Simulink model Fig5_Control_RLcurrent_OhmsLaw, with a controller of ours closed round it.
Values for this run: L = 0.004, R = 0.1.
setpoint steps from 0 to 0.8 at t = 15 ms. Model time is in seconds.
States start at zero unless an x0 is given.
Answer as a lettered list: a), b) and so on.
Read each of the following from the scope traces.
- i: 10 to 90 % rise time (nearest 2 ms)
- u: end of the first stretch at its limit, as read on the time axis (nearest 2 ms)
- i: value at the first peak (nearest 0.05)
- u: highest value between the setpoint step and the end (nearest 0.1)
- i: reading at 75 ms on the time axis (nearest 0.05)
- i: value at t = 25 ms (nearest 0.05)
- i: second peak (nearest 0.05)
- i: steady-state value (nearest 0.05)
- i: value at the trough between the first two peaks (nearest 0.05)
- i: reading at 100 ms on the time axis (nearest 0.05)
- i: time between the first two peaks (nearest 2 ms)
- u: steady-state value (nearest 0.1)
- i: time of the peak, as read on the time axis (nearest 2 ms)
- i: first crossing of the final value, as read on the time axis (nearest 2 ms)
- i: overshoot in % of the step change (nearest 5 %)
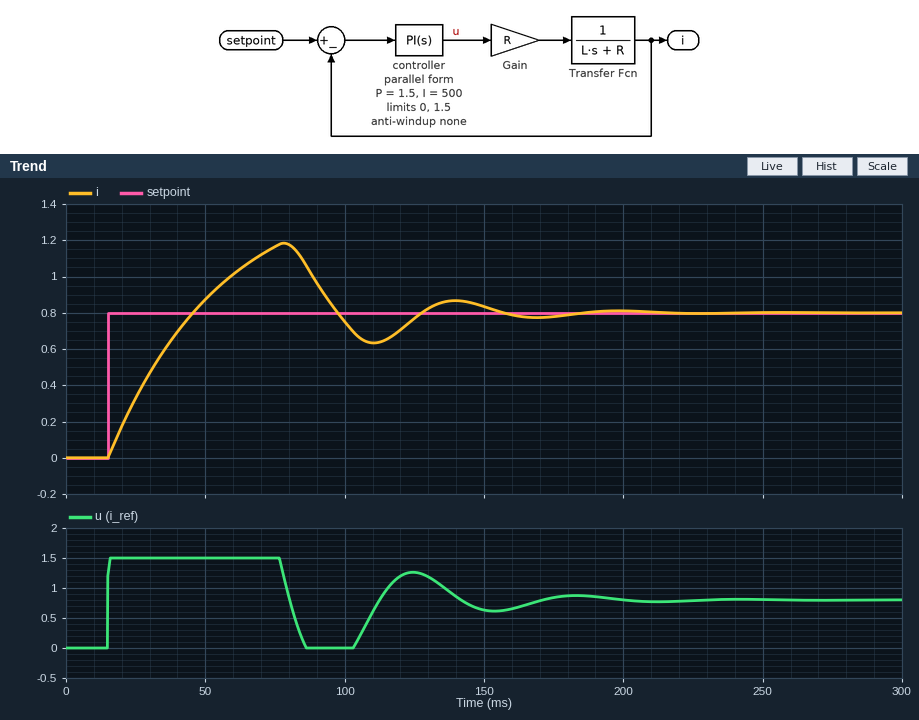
a) 24 ms
b) 76 ms
c) 1.20
d) 1.5
e) 1.15
f) 0.35
g) 0.85
h) 0.80
i) 0.65
j) 0.75
k) 62 ms
l) 0.8
m) 78 ms
n) 46 ms
o) 50 %
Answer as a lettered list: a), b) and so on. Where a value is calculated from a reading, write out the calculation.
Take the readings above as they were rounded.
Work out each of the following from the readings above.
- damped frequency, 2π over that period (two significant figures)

a) 2π / 62 = 0.10 rad/ms
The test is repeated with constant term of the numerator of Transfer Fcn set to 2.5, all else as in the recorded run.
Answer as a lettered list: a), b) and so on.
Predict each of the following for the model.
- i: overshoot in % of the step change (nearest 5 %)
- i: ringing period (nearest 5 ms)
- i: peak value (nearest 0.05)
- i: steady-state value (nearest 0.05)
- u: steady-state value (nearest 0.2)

a) 45 %
b) 45 ms
c) 1.15
d) 0.80
e) 0.4
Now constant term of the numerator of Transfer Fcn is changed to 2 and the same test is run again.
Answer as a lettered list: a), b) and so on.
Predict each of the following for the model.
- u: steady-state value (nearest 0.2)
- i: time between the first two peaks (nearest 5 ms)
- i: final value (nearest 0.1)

a) 0.4
b) 50 ms
c) 0.8
